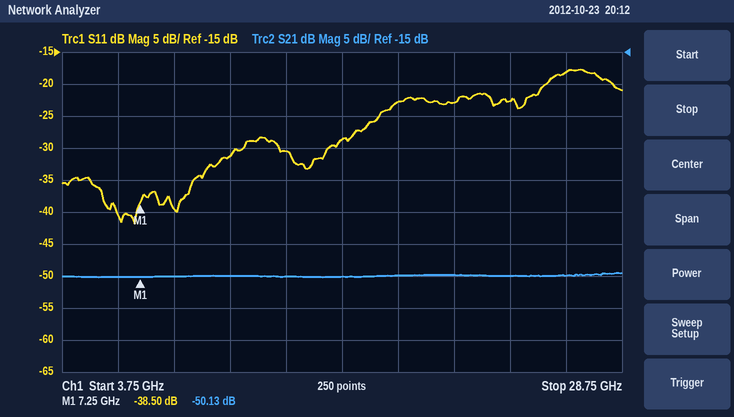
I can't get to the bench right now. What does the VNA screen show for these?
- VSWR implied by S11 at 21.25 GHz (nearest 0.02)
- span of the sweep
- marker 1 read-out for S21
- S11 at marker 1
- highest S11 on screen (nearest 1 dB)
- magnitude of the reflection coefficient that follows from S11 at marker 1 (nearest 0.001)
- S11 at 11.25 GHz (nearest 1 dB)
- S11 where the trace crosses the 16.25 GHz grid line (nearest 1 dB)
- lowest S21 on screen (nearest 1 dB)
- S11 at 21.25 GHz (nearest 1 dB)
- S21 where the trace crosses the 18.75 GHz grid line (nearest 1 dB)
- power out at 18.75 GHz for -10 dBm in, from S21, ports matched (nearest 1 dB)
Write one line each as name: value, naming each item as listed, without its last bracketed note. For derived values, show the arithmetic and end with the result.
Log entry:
VSWR implied by S11 at 21.25 GHz: |Γ| = 10^(-23/20) = 0.0708; VSWR = (1 + 0.0708)/(1 − 0.0708) ≈ 1.15, so 1.16 to the nearest 0.02
span of the sweep: 25 GHz
marker 1 read-out for S21: -50.13 dB
S11 at marker 1: -38.50 dB
highest S11 on screen: -18 dB
magnitude of the reflection coefficient that follows from S11 at marker 1: 10^(-38.5/20) ≈ 0.012
S11 at 11.25 GHz: -31 dB
S11 where the trace crosses the 16.25 GHz grid line: -29 dB
lowest S21 on screen: -50 dB
S11 at 21.25 GHz: -23 dB
S21 where the trace crosses the 18.75 GHz grid line: -50 dB
power out at 18.75 GHz for -10 dBm in, from S21, ports matched: -10 dBm + (-50 dB) = -60 dBm
